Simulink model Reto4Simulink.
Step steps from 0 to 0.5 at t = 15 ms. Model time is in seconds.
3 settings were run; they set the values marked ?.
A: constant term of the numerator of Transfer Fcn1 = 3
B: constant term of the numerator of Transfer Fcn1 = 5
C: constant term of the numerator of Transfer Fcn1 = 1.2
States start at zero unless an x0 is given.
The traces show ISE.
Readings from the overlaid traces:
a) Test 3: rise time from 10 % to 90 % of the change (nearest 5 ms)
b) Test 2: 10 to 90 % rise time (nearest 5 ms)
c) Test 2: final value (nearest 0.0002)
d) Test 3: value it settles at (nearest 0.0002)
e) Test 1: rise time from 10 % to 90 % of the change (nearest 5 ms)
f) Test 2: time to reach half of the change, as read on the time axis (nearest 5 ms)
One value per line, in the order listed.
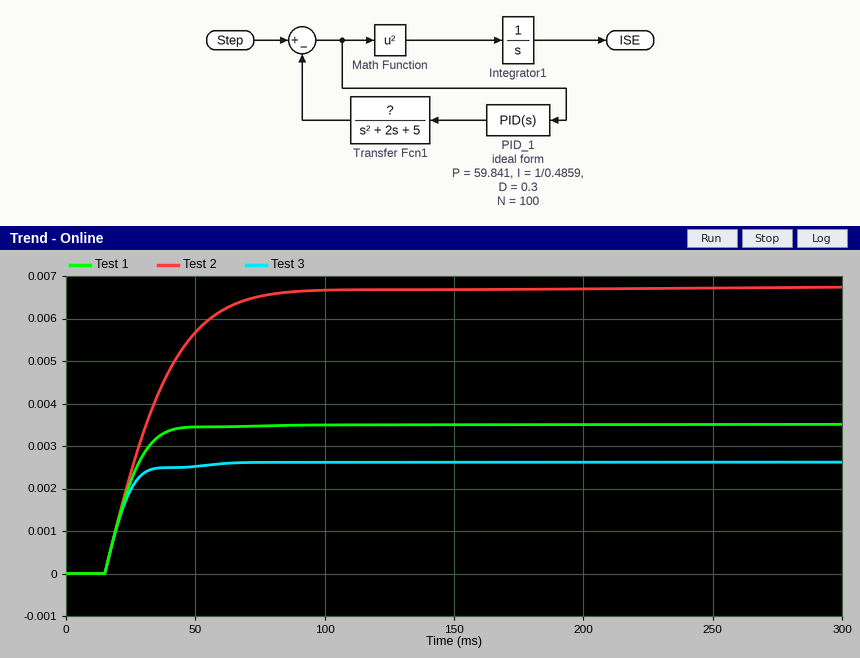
15 ms
40 ms
0.0068
0.0026
20 ms
30 ms
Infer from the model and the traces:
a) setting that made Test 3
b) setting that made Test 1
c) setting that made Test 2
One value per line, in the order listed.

B
A
C
